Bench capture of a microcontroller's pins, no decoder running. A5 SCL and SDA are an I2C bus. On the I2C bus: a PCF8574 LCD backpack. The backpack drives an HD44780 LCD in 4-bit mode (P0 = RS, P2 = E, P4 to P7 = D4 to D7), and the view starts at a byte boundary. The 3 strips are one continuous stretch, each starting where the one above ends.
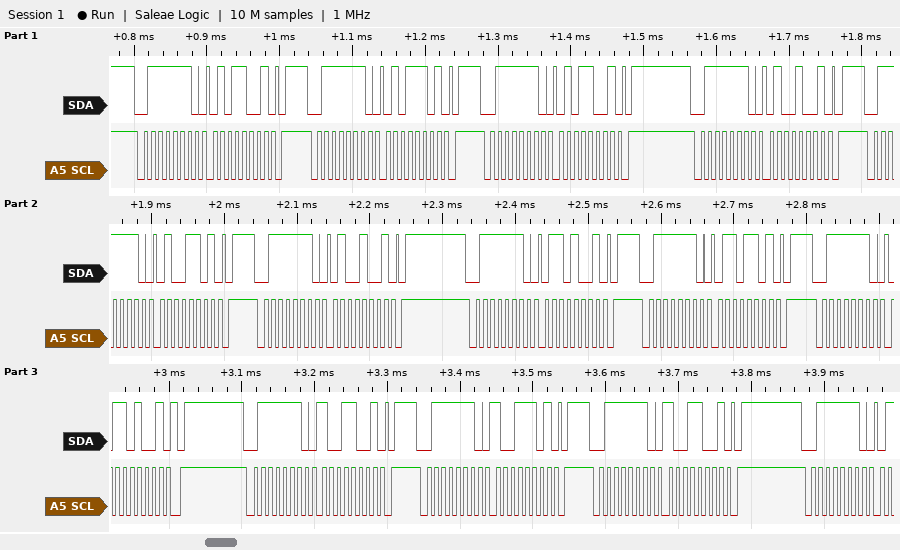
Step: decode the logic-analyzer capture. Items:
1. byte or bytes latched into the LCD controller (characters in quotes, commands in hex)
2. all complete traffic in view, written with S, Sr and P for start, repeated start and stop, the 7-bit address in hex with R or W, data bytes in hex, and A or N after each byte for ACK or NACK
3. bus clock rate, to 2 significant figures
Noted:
'T' 'i'
S 3FW A 59 A P S 3FW A 5D A P S 3FW A 59 A P S 3FW A 49 A P S 3FW A 4D A P S 3FW A 49 A P S 3FW A 69 A P S 3FW A 6D A P S 3FW A 69 A P S 3FW A 99 A P S 3FW A 9D A P S 3FW A 99 A P S 3FW A
100 kHz
